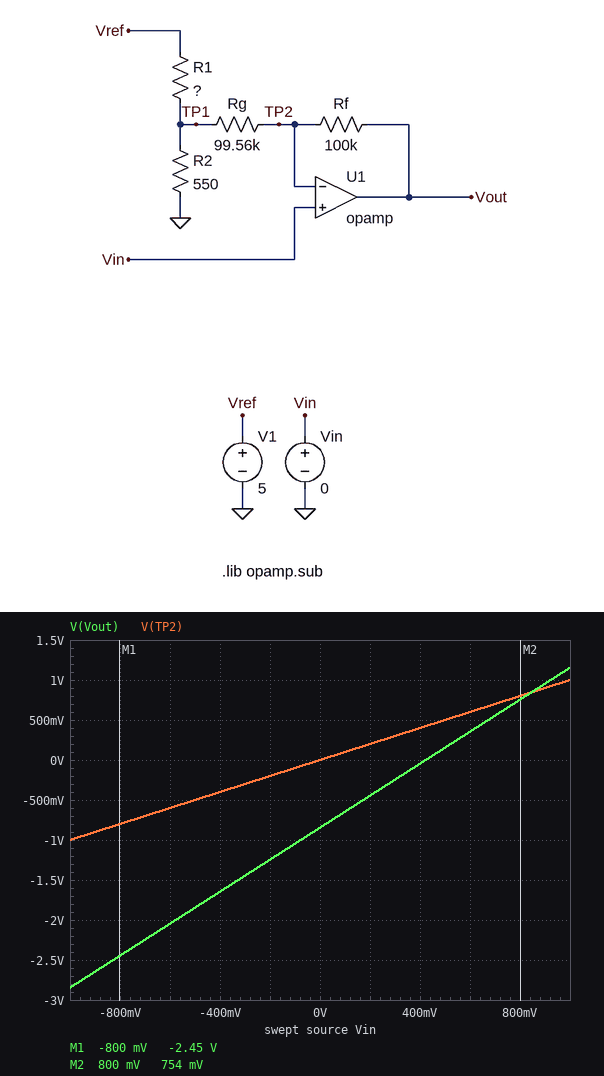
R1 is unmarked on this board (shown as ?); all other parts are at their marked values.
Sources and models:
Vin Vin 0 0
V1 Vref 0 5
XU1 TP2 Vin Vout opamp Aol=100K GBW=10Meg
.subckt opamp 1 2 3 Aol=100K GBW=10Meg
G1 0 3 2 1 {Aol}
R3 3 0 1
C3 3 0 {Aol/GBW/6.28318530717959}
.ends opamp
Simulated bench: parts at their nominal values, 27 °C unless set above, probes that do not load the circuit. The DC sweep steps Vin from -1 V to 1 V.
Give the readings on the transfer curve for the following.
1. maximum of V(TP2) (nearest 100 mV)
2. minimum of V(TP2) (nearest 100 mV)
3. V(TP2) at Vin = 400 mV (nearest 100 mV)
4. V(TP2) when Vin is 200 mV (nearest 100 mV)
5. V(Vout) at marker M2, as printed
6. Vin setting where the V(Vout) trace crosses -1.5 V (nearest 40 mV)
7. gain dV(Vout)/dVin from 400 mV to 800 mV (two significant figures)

1.0 V
-1.0 V
400 mV
200 mV
754 mV
-320 mV
2.0 V/V
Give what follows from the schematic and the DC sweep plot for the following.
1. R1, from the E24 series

2.7 kΩ
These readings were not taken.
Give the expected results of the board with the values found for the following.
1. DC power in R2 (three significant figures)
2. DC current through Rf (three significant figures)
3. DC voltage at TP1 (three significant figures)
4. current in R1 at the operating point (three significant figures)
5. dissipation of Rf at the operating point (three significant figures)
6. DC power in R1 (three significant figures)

1.29 mW
8.46 µA
842 mV
1.54 mA
7.16 µW
6.40 mW
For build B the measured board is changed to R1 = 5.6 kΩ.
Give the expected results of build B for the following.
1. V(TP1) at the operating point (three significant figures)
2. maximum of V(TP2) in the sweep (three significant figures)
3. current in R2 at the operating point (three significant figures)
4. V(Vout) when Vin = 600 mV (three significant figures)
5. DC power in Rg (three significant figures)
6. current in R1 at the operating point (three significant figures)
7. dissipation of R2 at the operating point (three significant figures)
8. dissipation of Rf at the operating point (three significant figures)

445 mV
1.00 V
809 µA
753 mV
1.99 µW
813 µA
360 µW
2.00 µW
